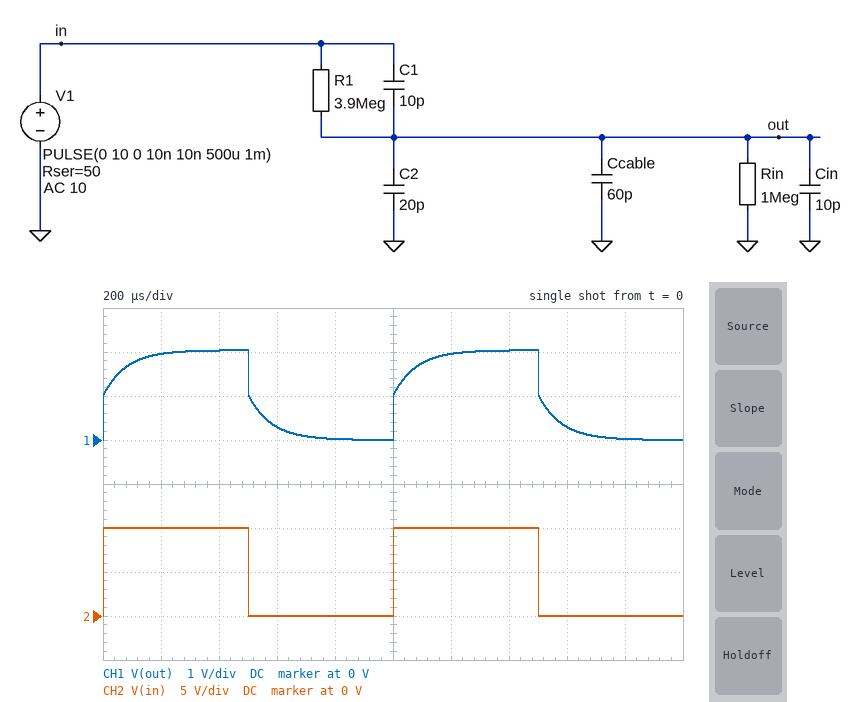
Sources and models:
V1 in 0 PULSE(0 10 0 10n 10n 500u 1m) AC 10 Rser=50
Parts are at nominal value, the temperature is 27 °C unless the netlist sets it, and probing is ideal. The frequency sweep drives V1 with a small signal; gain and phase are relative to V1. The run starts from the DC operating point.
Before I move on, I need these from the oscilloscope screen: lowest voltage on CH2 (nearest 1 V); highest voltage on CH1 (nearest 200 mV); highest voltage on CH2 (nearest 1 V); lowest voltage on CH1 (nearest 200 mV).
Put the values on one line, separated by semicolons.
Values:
0 V; 2.0 V; 10 V; 0 V
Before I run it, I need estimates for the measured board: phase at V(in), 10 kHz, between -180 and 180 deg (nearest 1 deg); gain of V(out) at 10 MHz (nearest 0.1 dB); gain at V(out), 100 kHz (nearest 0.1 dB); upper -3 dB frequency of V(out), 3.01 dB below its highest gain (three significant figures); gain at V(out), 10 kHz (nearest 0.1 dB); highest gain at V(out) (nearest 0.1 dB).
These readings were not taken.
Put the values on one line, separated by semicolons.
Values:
0 deg; -20.0 dB; -20.0 dB; 2.77 kHz; -19.5 dB; -13.8 dB
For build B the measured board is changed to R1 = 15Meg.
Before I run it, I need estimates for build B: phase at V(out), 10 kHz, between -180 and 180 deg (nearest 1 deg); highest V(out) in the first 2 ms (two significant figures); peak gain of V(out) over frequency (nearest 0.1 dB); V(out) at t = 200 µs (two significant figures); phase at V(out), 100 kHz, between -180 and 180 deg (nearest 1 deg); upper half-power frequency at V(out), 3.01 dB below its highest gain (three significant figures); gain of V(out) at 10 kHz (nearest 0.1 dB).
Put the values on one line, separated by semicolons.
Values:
4 deg; 1.0 V; -20.0 dB; 670 mV; 0 deg; 354 MHz; -20.1 dB
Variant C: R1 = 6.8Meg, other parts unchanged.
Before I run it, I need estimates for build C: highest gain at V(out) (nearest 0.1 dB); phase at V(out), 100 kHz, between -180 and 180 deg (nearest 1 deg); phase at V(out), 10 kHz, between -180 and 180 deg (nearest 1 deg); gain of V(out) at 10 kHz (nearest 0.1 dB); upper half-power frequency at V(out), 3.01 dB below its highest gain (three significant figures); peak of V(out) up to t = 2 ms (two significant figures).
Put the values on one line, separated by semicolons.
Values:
-17.8 dB; 0 deg; -3 deg; -19.9 dB; 165 MHz; 1.3 V
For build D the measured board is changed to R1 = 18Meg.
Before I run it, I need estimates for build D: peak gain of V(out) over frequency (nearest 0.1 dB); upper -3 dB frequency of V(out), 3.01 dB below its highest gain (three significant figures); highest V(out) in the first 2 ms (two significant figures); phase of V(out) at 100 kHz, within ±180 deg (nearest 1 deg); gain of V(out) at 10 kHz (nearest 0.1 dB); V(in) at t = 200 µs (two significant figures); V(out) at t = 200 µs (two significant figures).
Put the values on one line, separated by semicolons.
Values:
-20.0 dB; 354 MHz; 1.0 V; 0 deg; -20.1 dB; 10 V; 580 mV
